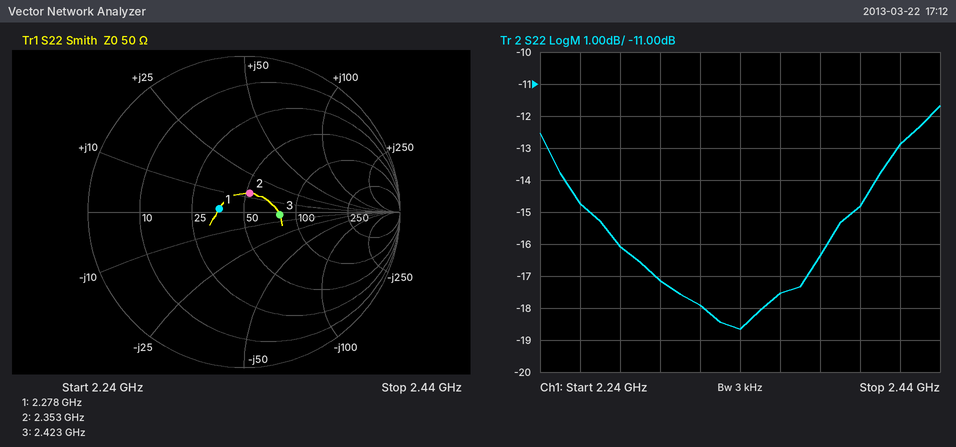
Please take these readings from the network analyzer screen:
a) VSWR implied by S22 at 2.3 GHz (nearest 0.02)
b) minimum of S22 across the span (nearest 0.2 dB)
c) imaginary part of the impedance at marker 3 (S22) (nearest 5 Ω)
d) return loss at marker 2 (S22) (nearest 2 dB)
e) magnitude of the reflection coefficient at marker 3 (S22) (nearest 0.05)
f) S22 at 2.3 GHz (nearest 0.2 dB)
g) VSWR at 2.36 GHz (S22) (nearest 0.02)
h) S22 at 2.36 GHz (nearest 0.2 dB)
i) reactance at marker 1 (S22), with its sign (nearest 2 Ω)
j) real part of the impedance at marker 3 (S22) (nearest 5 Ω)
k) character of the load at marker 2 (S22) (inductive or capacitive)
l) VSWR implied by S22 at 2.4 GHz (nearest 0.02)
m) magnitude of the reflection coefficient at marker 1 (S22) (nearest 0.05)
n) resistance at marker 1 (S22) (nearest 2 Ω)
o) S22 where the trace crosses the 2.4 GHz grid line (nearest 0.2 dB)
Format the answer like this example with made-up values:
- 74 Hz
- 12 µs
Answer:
- 1.32
- -18.6 dB
- -5 Ω
- 18 dB
- 0.25
- -17.2 dB
- 1.30
- -17.6 dB
- +2 Ω
- 80 Ω
- inductive
- 1.44
- 0.15
- 36 Ω
- -14.8 dB
